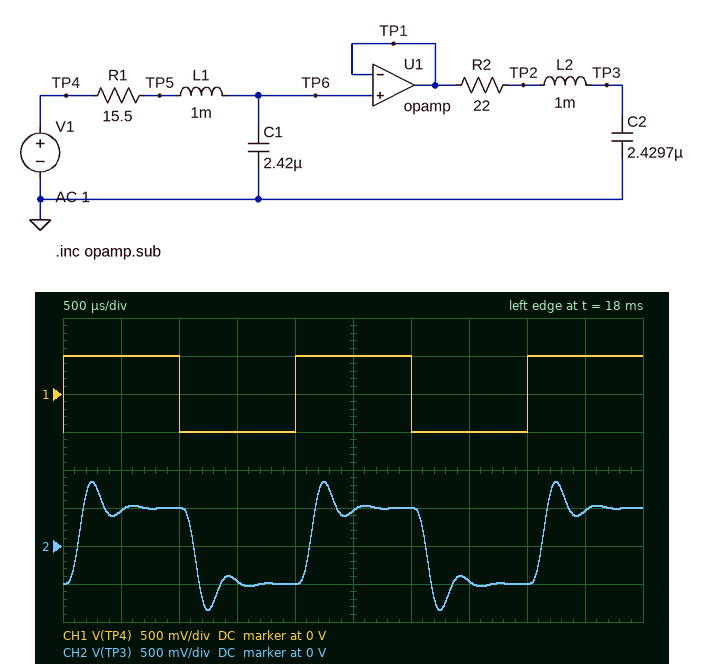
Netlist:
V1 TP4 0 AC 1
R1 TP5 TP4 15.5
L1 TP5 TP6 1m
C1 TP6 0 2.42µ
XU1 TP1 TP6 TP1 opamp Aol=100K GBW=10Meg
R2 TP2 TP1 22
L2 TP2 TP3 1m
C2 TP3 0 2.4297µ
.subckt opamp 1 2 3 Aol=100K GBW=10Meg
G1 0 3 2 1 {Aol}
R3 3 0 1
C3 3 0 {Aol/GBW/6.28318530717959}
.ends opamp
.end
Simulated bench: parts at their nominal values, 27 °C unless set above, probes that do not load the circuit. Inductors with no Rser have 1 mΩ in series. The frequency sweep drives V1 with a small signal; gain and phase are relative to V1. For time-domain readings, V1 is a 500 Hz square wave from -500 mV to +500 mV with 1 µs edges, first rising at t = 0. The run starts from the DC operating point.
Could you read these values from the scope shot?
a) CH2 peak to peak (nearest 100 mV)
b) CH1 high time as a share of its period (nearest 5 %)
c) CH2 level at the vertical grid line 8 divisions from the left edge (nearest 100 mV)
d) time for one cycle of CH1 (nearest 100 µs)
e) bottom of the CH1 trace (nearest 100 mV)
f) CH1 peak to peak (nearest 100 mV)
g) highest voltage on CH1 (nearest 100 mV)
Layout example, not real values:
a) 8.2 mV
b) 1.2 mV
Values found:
a) 1.7 V
b) 50 %
c) -500 mV
d) 2.0 ms
e) -500 mV
f) 1.0 V
g) 500 mV
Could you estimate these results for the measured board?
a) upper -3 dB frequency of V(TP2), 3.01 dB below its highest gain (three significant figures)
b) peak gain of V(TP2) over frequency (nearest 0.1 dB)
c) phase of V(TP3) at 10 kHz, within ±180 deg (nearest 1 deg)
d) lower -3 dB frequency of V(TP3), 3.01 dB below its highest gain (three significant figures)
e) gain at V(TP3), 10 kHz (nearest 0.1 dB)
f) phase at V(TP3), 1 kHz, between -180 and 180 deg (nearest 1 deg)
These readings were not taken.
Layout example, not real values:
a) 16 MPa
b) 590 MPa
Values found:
a) 2.34 kHz
b) 0 dB
c) 37 deg
d) 772 Hz
e) -38.3 dB
f) -35 deg
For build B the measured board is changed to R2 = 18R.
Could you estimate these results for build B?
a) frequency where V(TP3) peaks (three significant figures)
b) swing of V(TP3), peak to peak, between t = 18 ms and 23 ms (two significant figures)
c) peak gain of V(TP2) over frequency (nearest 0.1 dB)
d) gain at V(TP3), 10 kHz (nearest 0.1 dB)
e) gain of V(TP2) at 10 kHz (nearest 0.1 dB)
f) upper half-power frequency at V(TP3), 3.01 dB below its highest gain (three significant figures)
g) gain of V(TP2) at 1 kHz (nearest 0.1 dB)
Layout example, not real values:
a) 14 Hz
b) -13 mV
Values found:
a) 2.63 kHz
b) 1.9 V
c) 0.3 dB
d) -38.1 dB
e) -19.4 dB
f) 3.46 kHz
g) 0.2 dB
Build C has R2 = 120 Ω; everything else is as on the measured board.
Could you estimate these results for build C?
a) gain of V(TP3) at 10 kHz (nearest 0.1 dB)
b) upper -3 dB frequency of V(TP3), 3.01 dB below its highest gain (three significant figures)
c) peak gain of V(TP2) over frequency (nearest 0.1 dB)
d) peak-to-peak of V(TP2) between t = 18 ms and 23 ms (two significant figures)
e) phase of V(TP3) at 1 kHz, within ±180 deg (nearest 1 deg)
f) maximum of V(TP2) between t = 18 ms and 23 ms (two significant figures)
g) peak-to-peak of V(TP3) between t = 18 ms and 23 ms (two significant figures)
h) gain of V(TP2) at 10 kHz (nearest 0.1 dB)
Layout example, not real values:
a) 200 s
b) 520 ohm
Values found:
a) -45.1 dB
b) 588 Hz
c) 0 dB
d) 930 mV
e) -78 deg
f) 470 mV
g) 940 mV
h) -26.4 dB
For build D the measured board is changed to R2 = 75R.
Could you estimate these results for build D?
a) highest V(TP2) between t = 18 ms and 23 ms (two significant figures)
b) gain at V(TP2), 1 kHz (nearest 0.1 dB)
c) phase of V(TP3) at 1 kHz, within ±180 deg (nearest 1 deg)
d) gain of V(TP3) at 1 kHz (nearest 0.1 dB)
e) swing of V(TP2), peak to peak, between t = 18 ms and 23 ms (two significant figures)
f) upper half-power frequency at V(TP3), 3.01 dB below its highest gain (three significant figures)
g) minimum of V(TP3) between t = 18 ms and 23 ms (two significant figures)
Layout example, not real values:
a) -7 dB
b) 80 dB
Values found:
a) 500 mV
b) -3.6 dB
c) -66 deg
d) -2.7 dB
e) 990 mV
f) 1.09 kHz
g) -500 mV
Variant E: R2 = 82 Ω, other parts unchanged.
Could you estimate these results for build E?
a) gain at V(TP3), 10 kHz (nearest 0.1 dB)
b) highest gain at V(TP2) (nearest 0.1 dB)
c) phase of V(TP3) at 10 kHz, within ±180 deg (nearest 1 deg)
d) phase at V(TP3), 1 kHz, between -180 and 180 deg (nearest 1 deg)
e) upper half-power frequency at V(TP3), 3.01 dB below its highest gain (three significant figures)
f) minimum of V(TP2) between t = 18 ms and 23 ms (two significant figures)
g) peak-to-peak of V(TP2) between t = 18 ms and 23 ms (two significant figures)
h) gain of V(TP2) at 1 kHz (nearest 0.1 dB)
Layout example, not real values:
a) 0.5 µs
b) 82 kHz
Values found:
a) -42.6 dB
b) 0 dB
c) 71 deg
d) -69 deg
e) 955 Hz
f) -490 mV
g) 990 mV
h) -4.1 dB
